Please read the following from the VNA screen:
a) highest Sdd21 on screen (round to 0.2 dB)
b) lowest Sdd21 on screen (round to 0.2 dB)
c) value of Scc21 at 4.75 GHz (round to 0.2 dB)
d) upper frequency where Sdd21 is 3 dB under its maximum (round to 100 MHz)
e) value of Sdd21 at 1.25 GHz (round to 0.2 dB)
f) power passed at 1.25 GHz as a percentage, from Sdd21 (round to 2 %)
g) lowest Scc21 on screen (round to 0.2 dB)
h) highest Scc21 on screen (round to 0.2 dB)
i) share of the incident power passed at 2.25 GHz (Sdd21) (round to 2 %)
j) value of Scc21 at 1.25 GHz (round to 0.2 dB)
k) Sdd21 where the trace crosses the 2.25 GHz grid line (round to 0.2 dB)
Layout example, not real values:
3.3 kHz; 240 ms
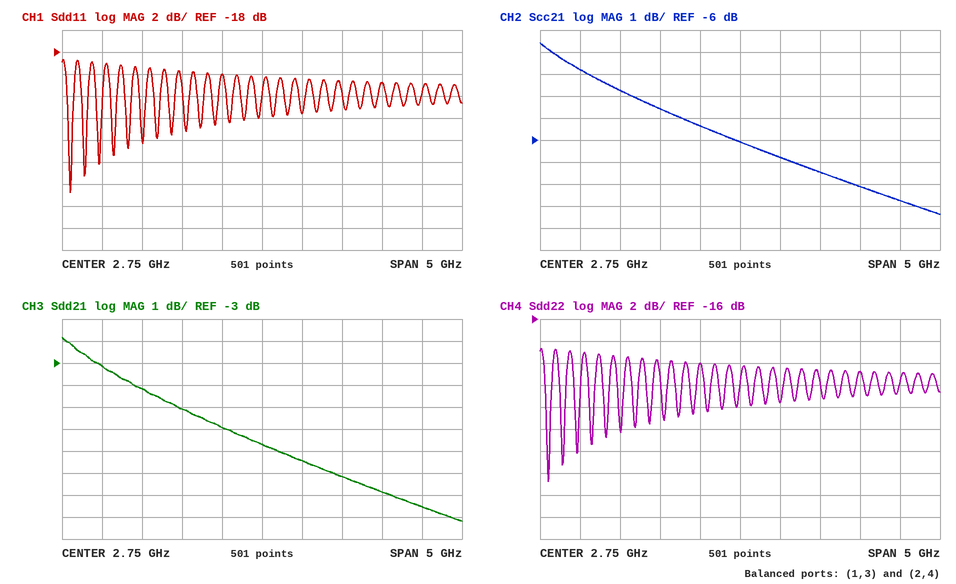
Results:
-1.8 dB; -10.2 dB; -8.8 dB; 1.6 GHz; -4.2 dB; 38 %; -9.4 dB; -1.6 dB; 26 %; -3.8 dB; -6.0 dB
